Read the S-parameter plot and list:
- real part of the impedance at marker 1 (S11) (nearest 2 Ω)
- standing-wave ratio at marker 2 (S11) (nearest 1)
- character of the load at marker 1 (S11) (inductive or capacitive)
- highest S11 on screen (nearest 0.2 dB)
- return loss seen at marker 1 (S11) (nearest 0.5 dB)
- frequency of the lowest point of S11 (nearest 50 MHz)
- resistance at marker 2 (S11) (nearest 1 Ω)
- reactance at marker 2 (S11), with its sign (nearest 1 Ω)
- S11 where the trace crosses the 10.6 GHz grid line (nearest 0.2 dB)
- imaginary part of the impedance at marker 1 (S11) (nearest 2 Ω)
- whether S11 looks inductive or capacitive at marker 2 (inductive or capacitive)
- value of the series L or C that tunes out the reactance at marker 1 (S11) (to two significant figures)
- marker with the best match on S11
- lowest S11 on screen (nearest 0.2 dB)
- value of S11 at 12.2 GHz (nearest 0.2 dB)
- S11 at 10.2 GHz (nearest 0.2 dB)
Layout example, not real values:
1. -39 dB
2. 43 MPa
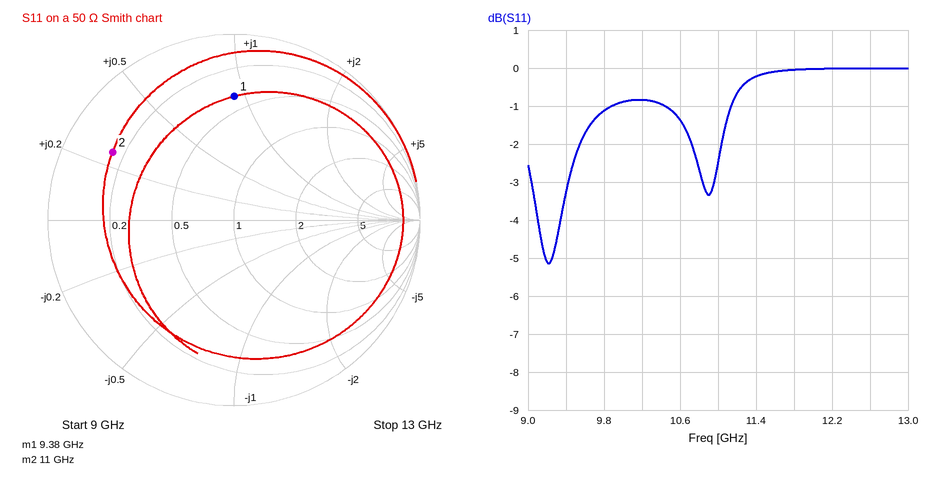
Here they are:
1. 20 Ω
2. 7
3. inductive
4. 0.0 dB
5. 3.5 dB
6. 9.20 GHz
7. 8 Ω
8. +13 Ω
9. -1.4 dB
10. +46 Ω
11. inductive
12. 370 fF
13. marker 1
14. -5.2 dB
15. 0.0 dB
16. -0.8 dB
